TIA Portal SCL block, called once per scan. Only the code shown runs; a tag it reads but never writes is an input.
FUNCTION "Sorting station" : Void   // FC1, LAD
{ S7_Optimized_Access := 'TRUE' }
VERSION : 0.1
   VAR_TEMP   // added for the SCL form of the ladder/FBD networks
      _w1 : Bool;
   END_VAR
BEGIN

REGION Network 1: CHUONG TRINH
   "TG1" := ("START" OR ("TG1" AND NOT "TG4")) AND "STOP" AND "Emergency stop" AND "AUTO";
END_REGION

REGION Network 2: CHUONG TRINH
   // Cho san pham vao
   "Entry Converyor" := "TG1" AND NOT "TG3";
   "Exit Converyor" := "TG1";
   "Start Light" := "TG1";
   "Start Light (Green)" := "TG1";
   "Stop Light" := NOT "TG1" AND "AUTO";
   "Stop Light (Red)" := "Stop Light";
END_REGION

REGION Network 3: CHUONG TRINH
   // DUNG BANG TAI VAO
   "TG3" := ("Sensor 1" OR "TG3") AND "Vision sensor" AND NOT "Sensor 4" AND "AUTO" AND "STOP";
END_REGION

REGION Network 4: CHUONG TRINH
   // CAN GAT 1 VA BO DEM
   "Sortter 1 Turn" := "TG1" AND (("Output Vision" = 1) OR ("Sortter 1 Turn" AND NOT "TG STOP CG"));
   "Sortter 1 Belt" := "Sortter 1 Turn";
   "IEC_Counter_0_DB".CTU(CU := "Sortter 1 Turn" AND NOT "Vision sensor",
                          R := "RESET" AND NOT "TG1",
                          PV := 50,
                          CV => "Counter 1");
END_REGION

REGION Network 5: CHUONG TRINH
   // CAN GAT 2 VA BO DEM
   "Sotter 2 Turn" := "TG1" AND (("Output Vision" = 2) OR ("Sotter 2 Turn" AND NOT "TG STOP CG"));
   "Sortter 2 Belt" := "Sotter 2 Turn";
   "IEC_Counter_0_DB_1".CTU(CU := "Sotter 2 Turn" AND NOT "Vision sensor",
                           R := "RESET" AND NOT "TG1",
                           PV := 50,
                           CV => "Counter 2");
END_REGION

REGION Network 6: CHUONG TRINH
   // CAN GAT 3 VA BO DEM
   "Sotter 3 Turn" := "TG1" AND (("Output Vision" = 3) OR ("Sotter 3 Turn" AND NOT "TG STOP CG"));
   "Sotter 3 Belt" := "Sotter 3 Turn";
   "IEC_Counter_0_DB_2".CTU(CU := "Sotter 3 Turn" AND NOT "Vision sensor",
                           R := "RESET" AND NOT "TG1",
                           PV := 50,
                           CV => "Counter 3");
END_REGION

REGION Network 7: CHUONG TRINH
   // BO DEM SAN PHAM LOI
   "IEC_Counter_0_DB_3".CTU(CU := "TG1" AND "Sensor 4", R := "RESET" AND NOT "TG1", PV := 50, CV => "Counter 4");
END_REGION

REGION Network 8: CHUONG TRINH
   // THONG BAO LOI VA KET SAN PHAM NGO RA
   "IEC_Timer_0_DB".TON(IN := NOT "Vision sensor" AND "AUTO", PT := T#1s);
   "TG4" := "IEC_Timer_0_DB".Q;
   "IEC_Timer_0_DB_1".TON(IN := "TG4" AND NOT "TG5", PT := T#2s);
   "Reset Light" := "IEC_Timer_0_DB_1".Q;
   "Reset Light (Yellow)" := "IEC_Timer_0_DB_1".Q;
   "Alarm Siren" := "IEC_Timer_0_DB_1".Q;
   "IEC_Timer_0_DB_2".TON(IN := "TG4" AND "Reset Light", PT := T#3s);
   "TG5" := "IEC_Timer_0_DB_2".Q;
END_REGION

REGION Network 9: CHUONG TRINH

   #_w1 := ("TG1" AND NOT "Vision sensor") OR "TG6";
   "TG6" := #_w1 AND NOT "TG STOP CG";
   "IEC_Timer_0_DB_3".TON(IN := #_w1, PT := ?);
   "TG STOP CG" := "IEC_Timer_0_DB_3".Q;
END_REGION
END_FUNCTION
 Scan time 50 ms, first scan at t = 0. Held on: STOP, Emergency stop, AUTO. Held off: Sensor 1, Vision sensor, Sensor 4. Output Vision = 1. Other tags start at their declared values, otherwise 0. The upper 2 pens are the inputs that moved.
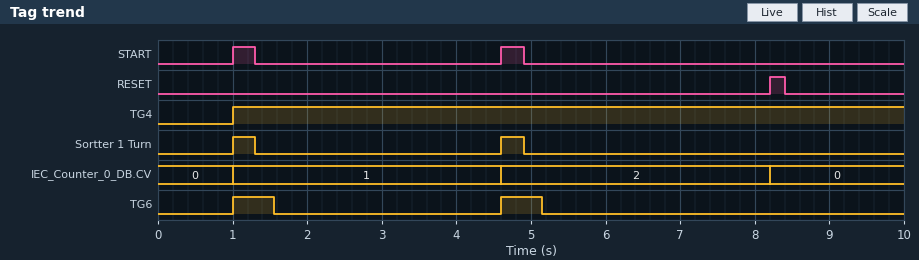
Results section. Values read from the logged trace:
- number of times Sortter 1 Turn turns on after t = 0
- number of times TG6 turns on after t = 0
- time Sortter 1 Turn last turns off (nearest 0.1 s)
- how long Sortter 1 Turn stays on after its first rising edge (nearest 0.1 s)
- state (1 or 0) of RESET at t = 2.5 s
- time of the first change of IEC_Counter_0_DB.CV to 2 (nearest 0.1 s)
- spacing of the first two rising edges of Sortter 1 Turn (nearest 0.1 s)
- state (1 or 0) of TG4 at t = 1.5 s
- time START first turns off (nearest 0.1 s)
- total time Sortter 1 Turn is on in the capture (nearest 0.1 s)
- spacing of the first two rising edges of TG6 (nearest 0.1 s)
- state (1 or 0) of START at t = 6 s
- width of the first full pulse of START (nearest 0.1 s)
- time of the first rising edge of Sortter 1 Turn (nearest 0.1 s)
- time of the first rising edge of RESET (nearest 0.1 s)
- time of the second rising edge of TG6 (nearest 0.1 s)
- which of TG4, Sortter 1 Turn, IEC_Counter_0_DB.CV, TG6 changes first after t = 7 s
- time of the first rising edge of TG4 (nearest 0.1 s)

2
2
4.9 s
0.3 s
0
4.6 s
3.6 s
1
1.3 s
0.6 s
3.6 s
0
0.3 s
1.0 s
8.2 s
4.6 s
IEC_Counter_0_DB.CV
1.0 s
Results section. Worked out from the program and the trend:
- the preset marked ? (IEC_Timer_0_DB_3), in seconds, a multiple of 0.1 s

0.5 s
